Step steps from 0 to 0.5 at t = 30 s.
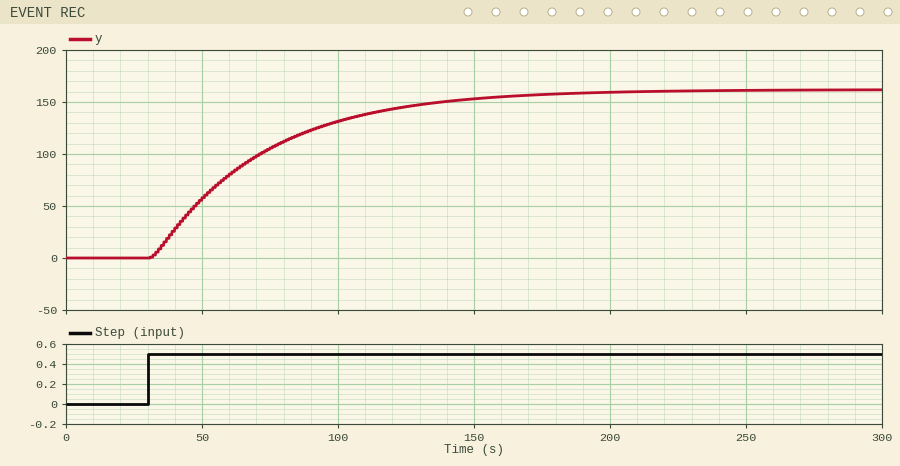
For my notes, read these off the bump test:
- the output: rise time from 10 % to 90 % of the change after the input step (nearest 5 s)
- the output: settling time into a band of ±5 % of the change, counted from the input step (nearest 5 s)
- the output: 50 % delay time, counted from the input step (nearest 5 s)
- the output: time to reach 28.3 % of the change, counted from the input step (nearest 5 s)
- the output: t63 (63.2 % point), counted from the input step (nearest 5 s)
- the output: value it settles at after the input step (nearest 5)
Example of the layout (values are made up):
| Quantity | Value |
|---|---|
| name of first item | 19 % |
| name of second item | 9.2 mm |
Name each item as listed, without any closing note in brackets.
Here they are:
| Quantity | Value |
|---|---|
| the output: rise time from 10 % to 90 % of the change after the input step | 90 s |
| the output: settling time into a band of ±5 % of the change, counted from the input step | 125 s |
| the output: 50 % delay time, counted from the input step | 30 s |
| the output: time to reach 28.3 % of the change, counted from the input step | 15 s |
| the output: t63 (63.2 % point), counted from the input step | 45 s |
| the output: value it settles at after the input step | 160 |
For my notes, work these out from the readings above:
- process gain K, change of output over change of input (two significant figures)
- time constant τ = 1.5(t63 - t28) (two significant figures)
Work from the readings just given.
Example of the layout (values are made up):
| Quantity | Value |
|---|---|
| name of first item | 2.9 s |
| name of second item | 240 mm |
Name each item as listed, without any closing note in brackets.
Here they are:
| Quantity | Value |
|---|---|
| process gain K, change of output over change of input | 320 |
| time constant τ = 1.5(t63 - t28) | 45 s |
